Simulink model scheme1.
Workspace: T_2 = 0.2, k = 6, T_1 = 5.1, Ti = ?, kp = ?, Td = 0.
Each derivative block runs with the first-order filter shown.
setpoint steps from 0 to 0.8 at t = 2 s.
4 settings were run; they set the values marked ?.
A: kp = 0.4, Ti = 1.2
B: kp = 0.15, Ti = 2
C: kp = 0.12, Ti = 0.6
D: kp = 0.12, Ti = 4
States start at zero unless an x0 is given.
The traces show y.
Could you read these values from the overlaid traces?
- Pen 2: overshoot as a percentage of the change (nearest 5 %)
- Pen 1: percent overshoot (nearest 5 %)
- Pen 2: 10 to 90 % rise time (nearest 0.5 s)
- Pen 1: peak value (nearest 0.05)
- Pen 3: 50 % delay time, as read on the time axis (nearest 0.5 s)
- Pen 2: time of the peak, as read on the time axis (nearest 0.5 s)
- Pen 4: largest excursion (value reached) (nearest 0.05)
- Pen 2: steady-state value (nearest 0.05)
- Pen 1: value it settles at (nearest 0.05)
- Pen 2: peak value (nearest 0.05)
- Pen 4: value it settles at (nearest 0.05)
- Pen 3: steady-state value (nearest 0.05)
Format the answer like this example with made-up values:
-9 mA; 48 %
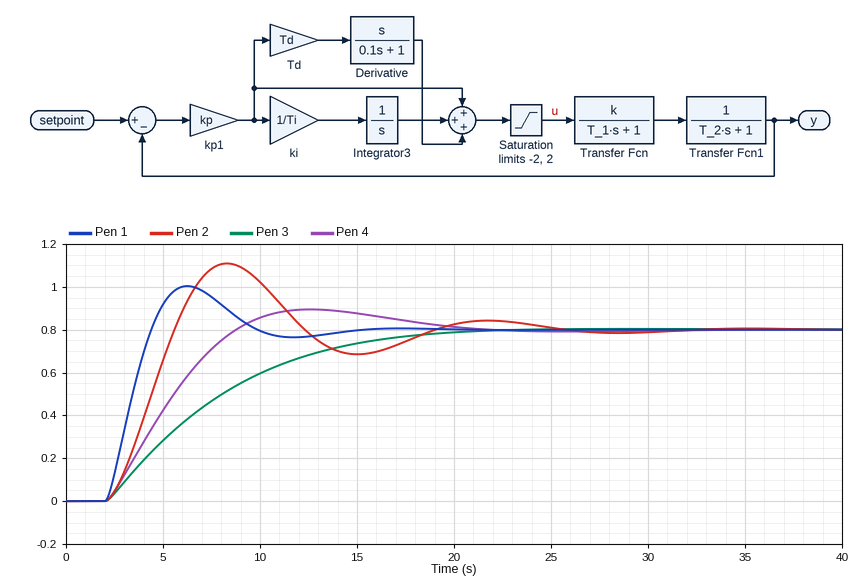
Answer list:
40 %; 25 %; 2.5 s; 1.00; 6.5 s; 8.5 s; 0.90; 0.80; 0.80; 1.10; 0.80; 0.80
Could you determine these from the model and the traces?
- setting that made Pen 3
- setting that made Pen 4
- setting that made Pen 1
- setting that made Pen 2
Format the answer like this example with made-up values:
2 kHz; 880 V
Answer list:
D; B; A; C
